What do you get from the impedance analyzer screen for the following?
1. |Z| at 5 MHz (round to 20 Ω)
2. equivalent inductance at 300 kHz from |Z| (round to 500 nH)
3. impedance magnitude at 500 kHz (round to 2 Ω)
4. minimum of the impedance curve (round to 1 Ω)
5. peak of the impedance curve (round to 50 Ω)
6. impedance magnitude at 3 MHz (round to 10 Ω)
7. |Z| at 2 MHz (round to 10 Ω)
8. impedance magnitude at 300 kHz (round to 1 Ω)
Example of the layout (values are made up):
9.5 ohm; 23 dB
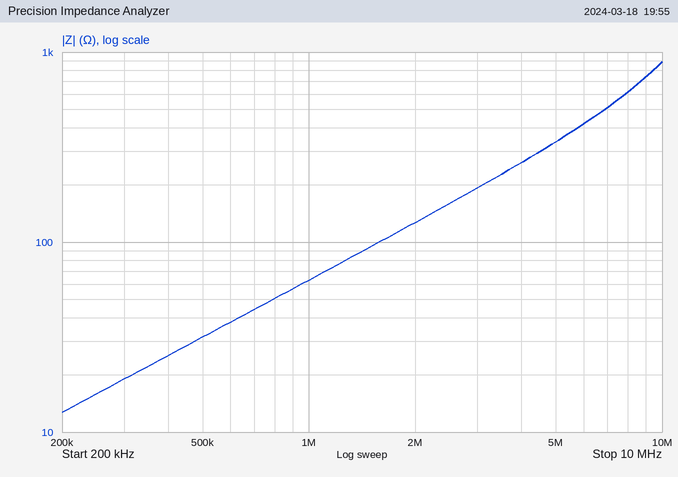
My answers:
340 Ω; 10.0 µH; 32 Ω; 13 Ω; 900 Ω; 190 Ω; 130 Ω; 19 Ω
